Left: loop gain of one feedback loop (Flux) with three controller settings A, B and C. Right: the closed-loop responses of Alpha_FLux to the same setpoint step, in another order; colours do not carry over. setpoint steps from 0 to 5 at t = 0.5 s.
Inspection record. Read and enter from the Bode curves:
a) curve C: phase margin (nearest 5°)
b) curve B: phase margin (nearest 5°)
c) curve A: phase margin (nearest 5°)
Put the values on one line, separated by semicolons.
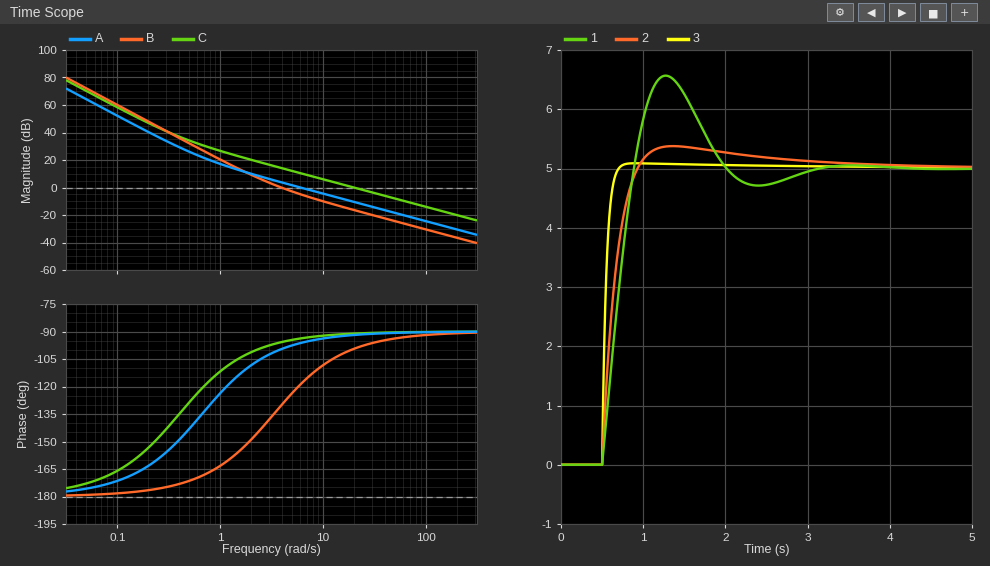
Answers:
90°; 50°; 85°
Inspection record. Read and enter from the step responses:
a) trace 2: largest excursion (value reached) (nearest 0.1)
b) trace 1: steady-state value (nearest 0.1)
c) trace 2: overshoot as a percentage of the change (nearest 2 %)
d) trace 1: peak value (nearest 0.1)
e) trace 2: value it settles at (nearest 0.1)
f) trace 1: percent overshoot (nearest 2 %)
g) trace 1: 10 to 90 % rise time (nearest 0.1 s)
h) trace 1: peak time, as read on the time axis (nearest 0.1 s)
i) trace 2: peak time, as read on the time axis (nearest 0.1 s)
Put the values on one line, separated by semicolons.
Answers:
5.4; 5.0; 8 %; 6.6; 5.0; 32 %; 0.3 s; 1.3 s; 1.4 s
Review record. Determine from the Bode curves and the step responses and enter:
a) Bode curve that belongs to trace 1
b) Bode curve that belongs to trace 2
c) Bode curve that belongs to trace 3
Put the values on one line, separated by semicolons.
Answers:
B; A; C
